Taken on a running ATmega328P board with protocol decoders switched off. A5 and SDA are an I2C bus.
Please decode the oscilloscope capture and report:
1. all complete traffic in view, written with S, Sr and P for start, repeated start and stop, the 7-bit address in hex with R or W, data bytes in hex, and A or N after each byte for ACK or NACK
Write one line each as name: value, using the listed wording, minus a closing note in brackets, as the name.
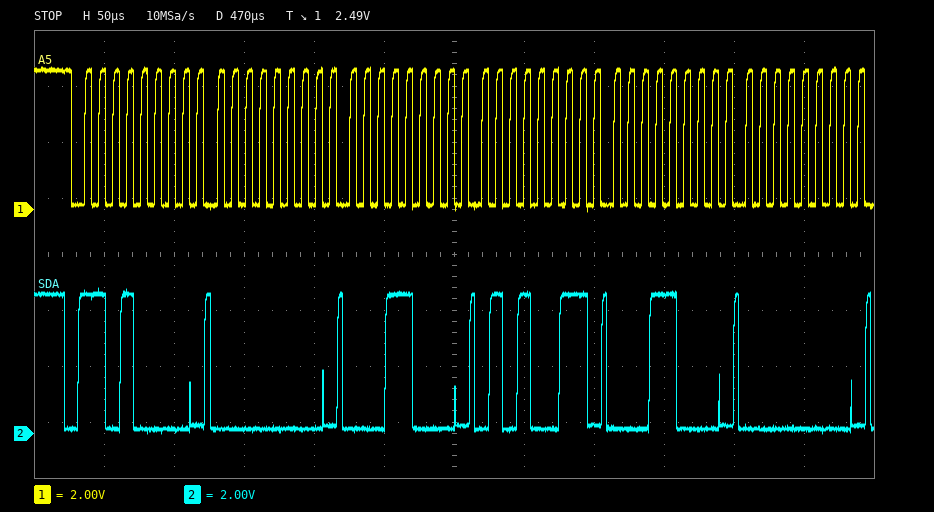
all complete traffic in view, written with S, Sr and P for start, repeated start and stop, the 7-bit address in hex with R or W, data bytes in hex, and A or N after each byte for ACK or NACK: S 68W A 00 A 18 A 53 A 18 A 00 A
